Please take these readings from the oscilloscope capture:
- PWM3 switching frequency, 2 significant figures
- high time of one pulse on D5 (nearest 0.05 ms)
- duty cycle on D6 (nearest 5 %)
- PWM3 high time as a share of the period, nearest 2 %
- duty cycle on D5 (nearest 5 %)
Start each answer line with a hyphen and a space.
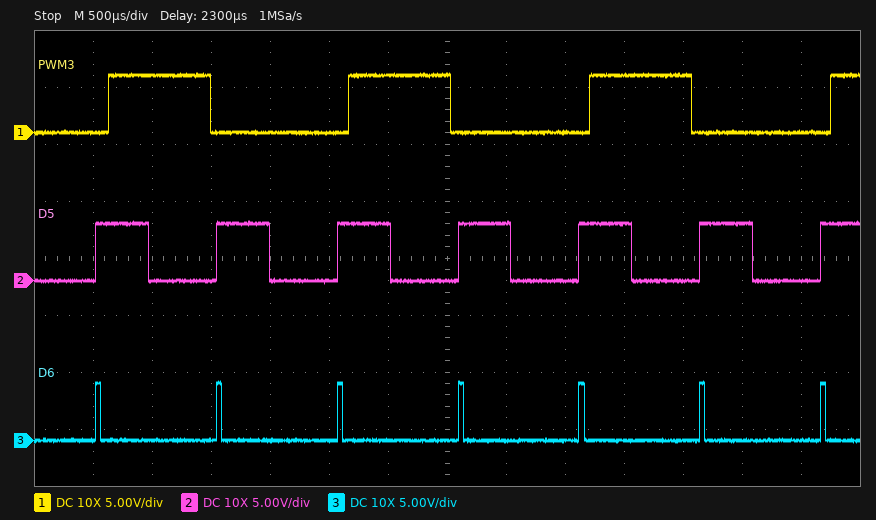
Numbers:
- 490 Hz
- 0.45 ms
- 5 %
- 42 %
- 45 %
